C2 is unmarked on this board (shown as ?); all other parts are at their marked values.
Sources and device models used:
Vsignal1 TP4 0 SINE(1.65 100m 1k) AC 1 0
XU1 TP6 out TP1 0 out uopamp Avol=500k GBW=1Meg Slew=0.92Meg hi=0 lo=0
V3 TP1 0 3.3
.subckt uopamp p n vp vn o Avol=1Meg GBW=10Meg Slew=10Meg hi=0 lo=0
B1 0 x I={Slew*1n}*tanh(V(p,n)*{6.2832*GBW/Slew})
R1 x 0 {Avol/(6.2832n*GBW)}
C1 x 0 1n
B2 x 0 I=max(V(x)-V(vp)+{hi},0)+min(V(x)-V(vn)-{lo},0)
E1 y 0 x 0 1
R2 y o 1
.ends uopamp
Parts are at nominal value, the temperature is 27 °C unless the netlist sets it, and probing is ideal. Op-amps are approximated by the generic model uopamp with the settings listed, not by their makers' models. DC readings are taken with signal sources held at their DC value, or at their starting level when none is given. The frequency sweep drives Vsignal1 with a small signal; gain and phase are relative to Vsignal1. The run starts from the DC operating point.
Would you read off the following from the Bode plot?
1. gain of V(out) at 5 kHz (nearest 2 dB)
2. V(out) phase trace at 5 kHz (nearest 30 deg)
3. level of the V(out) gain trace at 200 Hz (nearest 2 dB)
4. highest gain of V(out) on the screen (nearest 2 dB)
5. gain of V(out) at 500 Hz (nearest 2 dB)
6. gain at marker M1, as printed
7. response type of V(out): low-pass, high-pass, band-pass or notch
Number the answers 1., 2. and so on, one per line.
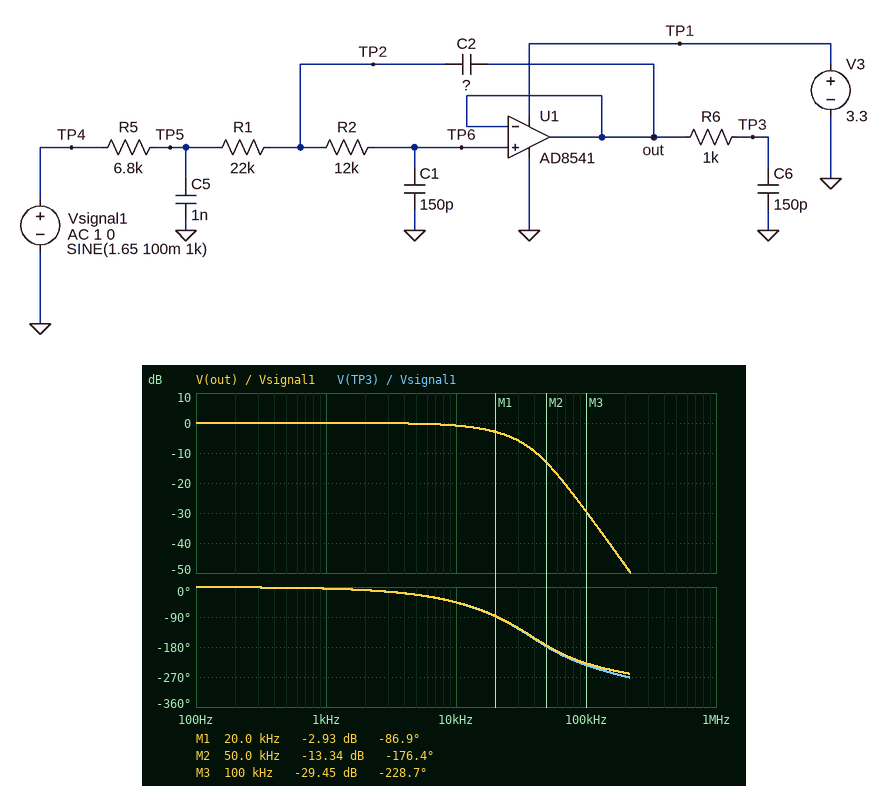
1. 0 dB
2. -30 deg
3. 0 dB
4. 0 dB
5. 0 dB
6. -2.93 dB
7. low-pass
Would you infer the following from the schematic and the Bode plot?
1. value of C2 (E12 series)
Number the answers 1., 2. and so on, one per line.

1. 390 pF
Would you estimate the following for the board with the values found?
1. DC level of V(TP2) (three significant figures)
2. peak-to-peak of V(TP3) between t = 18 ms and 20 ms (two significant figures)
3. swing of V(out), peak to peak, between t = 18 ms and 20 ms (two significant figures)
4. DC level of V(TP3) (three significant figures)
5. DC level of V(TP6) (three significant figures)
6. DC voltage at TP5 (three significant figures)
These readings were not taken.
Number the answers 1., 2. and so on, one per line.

1. 1.65 V
2. 200 mV
3. 200 mV
4. 1.65 V
5. 1.65 V
6. 1.65 V
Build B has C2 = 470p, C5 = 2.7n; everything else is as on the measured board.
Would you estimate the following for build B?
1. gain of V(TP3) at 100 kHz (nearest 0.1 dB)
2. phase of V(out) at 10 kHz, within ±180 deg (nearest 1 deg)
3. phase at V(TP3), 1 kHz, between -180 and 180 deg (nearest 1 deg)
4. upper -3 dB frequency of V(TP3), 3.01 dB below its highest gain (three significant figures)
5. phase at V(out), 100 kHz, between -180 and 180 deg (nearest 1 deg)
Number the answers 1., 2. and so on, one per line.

1. -39.2 dB
2. -71 deg
3. -9 deg
4. 8.51 kHz
5. 116 deg
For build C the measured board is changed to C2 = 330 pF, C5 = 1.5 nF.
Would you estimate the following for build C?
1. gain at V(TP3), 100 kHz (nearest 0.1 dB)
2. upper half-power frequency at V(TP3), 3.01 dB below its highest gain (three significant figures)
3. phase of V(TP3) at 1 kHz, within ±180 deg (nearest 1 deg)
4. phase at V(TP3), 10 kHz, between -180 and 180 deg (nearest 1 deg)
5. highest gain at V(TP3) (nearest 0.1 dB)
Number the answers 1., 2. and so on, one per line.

1. -31.5 dB
2. 14.0 kHz
3. -6 deg
4. -55 deg
5. 0 dB
